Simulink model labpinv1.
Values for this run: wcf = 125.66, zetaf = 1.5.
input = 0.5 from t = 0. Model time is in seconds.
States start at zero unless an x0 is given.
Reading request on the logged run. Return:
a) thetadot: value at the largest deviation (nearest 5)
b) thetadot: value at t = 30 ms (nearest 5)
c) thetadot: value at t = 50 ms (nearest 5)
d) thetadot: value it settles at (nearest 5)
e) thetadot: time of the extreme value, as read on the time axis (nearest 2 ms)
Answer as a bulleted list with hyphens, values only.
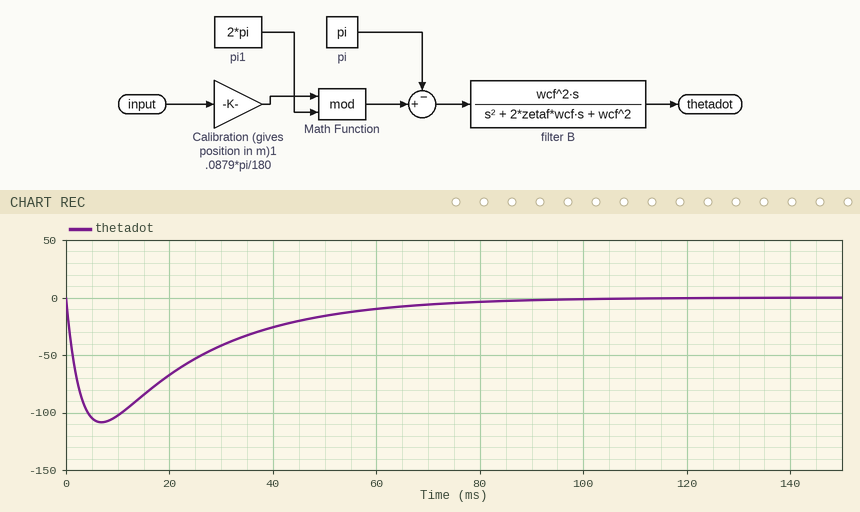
- -110
- -40
- -15
- 0
- 6 ms
